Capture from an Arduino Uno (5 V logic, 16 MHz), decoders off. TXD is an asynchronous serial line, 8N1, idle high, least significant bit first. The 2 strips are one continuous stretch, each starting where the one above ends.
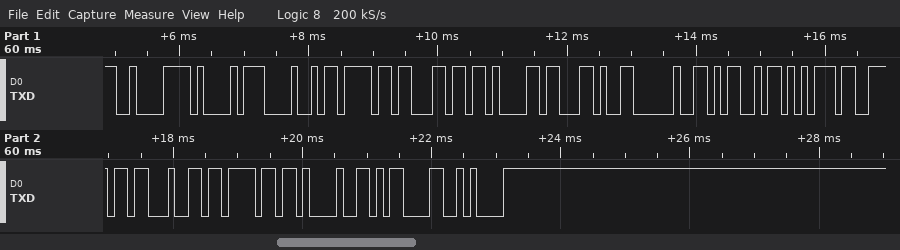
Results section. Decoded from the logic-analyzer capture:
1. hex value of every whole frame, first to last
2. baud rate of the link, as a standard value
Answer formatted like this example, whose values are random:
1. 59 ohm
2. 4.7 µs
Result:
1. 0xC2 0xA1 0x48 0x6F 0x6C 0x61 0x2C 0x20 0x4D 0x75 0x6E 0x64 0x6F 0x21 0x0D 0x0A
2. 9600 baud
